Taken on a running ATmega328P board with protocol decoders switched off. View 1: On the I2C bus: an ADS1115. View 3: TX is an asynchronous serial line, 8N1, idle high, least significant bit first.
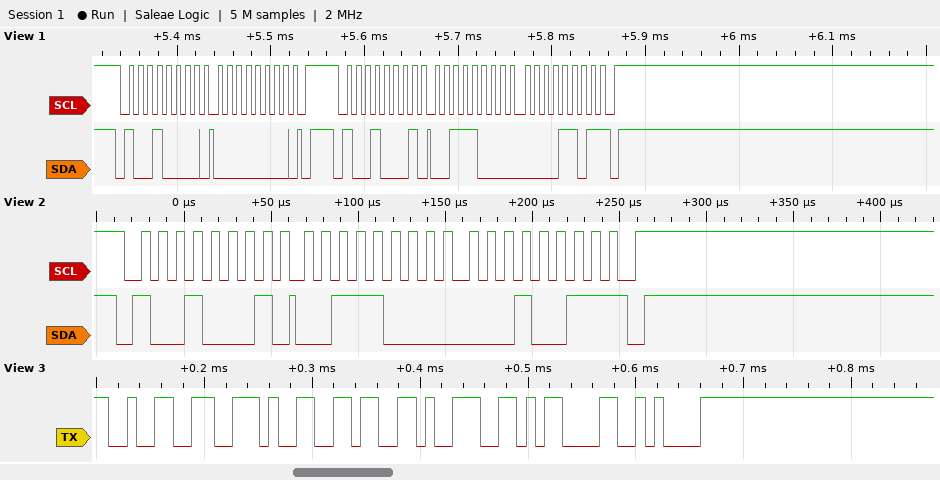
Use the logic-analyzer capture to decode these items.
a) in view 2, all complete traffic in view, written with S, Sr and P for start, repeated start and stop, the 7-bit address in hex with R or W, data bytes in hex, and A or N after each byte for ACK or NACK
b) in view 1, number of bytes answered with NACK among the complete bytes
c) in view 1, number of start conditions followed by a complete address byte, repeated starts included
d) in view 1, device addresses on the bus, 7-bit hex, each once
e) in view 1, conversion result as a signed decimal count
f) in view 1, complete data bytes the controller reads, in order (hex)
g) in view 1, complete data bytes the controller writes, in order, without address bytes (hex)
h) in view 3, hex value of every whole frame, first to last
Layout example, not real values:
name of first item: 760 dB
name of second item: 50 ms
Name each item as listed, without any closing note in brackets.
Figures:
in view 2, all complete traffic in view, written with S, Sr and P for start, repeated start and stop, the 7-bit address in hex with R or W, data bytes in hex, and A or N after each byte for ACK or NACK: S 48R A 38 A 13 N P
in view 1, number of bytes answered with NACK among the complete bytes: 1
in view 1, number of start conditions followed by a complete address byte, repeated starts included: 2
in view 1, device addresses on the bus, 7-bit hex, each once: 0x48
in view 1, conversion result as a signed decimal count: 14349
in view 1, complete data bytes the controller reads, in order: 38 0D
in view 1, complete data bytes the controller writes, in order, without address bytes: 00
in view 3, hex value of every whole frame, first to last: 32 2E 36 39 0D 0A
